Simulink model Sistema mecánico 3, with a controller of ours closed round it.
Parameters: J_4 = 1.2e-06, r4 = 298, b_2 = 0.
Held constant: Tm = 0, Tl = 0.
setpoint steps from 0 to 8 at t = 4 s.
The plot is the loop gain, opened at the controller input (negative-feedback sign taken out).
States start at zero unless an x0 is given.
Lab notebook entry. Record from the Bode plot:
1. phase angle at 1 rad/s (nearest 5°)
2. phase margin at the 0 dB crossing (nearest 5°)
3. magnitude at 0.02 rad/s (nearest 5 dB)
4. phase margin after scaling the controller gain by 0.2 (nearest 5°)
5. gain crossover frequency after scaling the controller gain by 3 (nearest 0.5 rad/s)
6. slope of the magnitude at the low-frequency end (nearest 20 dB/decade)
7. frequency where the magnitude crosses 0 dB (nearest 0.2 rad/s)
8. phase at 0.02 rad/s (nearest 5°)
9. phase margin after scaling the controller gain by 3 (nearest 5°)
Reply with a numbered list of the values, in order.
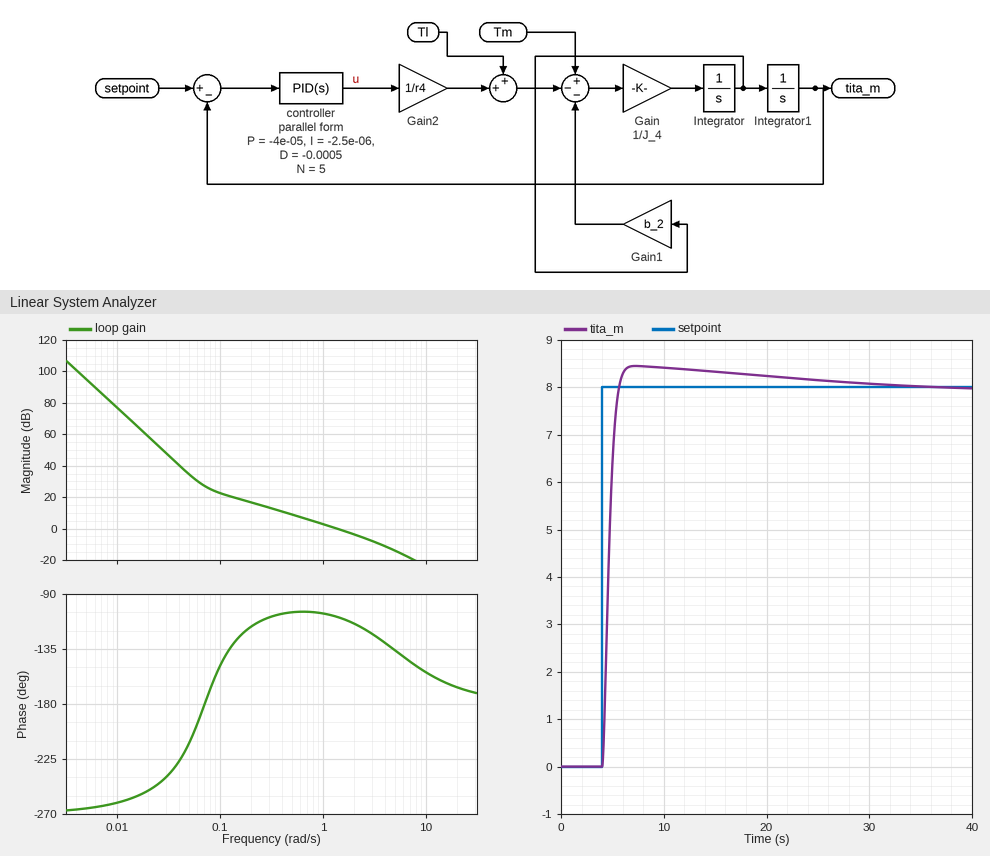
1. -105°
2. 70°
3. 60 dB
4. 70°
5. 3.5 rad/s
6. -60 dB/decade
7. 1.4 rad/s
8. -250°
9. 55°
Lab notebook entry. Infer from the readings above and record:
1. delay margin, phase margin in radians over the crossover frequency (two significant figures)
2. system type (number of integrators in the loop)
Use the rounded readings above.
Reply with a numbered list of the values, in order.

1. 0.87 s
2. 3
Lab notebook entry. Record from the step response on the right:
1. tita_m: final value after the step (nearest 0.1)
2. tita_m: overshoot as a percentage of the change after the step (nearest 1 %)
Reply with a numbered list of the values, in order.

1. 8.0
2. 6 %
